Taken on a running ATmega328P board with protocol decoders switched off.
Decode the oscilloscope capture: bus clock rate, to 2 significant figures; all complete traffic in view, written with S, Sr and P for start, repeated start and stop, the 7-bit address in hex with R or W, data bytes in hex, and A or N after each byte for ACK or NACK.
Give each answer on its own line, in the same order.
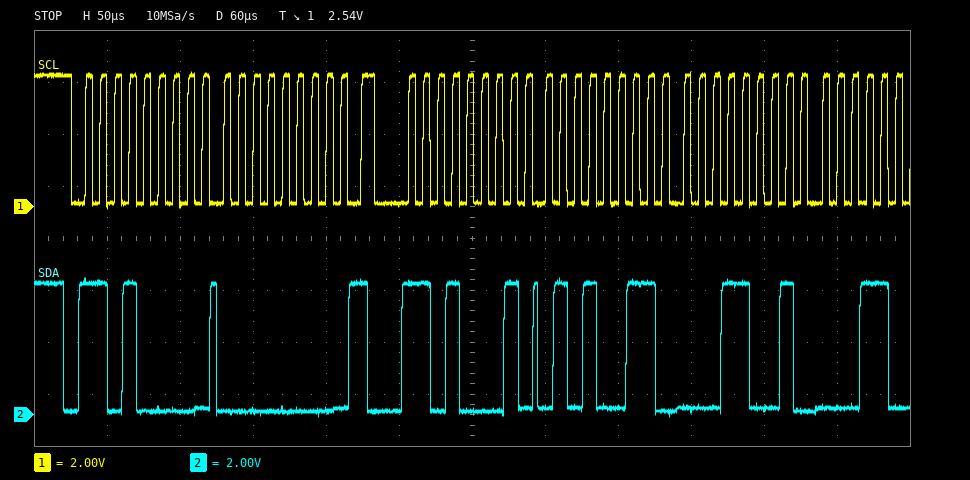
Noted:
100 kHz
S 68W A 00 A Sr 68R A 53 A 19 A
